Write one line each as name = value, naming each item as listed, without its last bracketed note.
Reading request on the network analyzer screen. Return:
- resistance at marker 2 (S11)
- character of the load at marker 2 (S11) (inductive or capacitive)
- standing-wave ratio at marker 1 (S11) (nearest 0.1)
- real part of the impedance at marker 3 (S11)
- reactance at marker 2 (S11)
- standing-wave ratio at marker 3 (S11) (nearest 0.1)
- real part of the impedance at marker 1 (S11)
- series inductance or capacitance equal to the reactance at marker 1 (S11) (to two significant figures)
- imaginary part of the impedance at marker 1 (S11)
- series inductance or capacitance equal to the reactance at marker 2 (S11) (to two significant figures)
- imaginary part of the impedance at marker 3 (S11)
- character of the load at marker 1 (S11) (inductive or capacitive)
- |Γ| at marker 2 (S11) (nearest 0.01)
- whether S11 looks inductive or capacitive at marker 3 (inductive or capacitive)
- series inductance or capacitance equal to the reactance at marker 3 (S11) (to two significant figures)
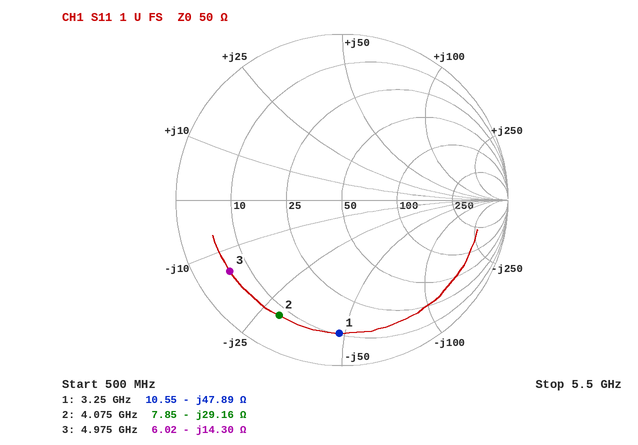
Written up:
resistance at marker 2 = 7.85 Ω
character of the load at marker 2 (S11) = capacitive
standing-wave ratio at marker 1 (S11) = 9.2
real part of the impedance at marker 3 = 6.02 Ω
reactance at marker 2 = -29.16 Ω
standing-wave ratio at marker 3 (S11) = 9.0
real part of the impedance at marker 1 = 10.55 Ω
series inductance or capacitance equal to the reactance at marker 1 (S11) = 1.0 pF
imaginary part of the impedance at marker 1 = -47.89 Ω
series inductance or capacitance equal to the reactance at marker 2 (S11) = 1.3 pF
imaginary part of the impedance at marker 3 = -14.30 Ω
character of the load at marker 1 (S11) = capacitive
|Γ| at marker 2 (S11) = 0.79
whether S11 looks inductive or capacitive at marker 3 = capacitive
series inductance or capacitance equal to the reactance at marker 3 (S11) = 2.2 pF
